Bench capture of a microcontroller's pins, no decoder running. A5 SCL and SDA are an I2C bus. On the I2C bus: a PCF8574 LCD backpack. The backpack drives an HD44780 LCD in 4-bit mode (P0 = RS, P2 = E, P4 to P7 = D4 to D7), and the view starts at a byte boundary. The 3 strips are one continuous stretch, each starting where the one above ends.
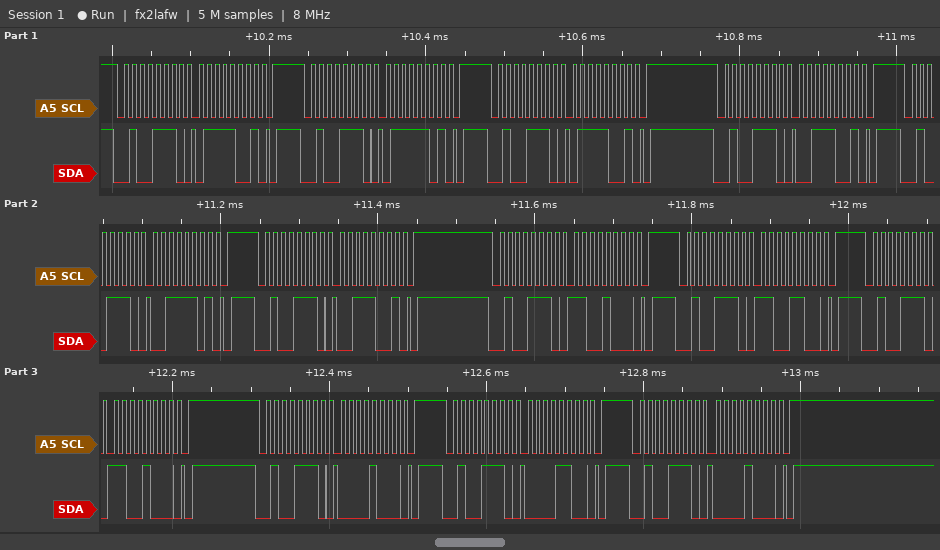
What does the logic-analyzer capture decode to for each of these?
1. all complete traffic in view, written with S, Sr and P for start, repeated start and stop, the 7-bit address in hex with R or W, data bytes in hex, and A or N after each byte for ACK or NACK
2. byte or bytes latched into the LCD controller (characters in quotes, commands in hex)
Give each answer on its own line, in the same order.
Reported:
S 27W A 79 A P S 27W A 7D A P S 27W A 79 A P S 27W A 39 A P S 27W A 3D A P S 27W A 39 A P S 27W A C8 A P S 27W A CC A P S 27W A C8 A P S 27W A 08 A P S 27W A 0C A P S 27W A 08 A P
's' 0xC0
